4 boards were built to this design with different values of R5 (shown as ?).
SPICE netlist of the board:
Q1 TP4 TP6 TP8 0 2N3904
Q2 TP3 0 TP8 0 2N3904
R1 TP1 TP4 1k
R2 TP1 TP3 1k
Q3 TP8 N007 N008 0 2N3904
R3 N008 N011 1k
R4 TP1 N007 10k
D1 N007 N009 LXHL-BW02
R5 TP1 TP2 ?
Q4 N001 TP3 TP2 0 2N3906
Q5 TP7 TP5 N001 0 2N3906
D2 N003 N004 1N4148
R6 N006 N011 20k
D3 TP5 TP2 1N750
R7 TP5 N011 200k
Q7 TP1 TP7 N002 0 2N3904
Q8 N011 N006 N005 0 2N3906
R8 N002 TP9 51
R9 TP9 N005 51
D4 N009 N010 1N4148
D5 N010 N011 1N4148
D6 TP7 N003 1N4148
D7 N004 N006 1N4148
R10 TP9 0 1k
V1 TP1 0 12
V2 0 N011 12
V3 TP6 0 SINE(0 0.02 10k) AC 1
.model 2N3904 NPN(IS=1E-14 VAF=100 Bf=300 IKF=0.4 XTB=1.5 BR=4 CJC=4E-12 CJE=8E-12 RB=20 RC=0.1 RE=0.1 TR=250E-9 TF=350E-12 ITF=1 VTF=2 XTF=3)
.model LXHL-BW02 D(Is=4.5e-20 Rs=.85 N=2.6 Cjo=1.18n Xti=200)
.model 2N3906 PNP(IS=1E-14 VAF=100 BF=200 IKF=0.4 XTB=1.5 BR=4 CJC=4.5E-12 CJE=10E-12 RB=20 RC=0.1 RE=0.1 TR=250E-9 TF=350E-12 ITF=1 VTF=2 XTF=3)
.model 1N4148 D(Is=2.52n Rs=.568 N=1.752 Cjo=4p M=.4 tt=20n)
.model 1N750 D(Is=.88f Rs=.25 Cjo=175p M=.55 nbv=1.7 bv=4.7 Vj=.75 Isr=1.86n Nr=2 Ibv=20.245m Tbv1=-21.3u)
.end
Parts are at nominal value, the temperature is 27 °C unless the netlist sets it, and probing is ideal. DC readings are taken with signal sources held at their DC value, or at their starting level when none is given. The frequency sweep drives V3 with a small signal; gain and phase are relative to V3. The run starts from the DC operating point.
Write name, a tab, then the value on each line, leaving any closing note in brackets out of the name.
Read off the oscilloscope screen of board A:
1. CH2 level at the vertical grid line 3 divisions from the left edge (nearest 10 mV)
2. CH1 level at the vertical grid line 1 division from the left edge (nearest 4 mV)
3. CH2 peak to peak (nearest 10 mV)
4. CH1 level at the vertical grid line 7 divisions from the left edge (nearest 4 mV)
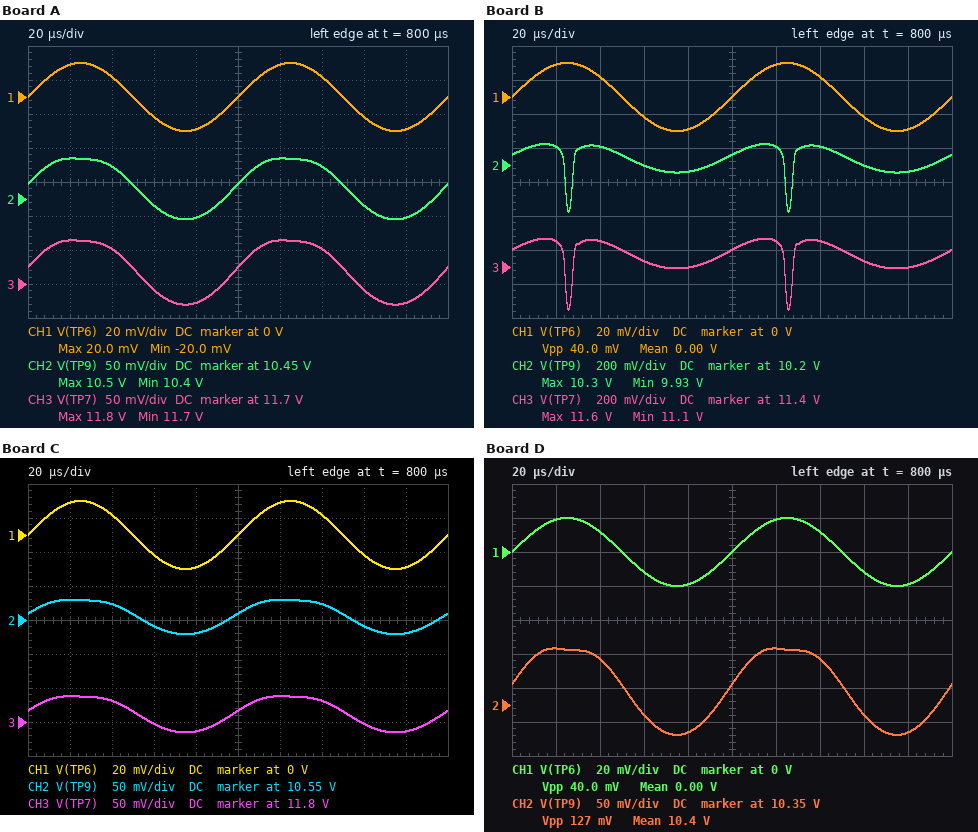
CH2 level at the vertical grid line 3 divisions from the left edge	10.44 V
CH1 level at the vertical grid line 1 division from the left edge	20 mV
CH2 peak to peak	90 mV
CH1 level at the vertical grid line 7 divisions from the left edge	12 mV
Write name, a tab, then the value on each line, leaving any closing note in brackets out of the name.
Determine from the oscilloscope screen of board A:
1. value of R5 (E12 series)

value of R5	120 Ω
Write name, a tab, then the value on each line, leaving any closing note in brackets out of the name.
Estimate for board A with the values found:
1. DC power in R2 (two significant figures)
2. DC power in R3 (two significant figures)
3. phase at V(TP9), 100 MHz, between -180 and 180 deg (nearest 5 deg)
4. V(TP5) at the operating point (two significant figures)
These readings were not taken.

DC power in R2	870 µW
DC power in R3	9.8 mW
phase at V(TP9), 100 MHz, between -180 and 180 deg	-60 deg
V(TP5) at the operating point	11 V
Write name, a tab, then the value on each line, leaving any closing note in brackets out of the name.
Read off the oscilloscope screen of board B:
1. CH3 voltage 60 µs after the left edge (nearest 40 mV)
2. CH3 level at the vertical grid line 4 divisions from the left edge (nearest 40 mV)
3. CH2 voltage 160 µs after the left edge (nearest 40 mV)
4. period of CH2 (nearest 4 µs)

CH3 voltage 60 µs after the left edge	11.44 V
CH3 level at the vertical grid line 4 divisions from the left edge	11.40 V
CH2 voltage 160 µs after the left edge	10.20 V
period of CH2	100 µs
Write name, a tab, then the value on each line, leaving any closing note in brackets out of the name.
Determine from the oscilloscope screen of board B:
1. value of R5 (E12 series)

value of R5	270 Ω
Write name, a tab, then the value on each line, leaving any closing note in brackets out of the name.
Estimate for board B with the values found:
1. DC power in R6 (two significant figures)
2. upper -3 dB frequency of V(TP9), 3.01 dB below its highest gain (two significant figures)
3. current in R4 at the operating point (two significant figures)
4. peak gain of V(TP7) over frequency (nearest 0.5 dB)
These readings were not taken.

DC power in R6	24 mW
upper -3 dB frequency of V(TP9), 3.01 dB below its highest gain	47 MHz
current in R4 at the operating point	2.0 mA
peak gain of V(TP7) over frequency	16.0 dB
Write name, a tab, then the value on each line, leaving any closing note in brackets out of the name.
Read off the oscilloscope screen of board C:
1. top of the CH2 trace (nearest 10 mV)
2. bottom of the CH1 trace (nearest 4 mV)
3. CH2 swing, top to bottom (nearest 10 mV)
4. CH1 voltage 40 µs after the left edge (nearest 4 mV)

top of the CH2 trace	10.58 V
bottom of the CH1 trace	-20 mV
CH2 swing, top to bottom	50 mV
CH1 voltage 40 µs after the left edge	12 mV
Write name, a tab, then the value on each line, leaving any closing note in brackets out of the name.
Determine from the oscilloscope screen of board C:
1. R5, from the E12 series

R5, from the E12 series	68 Ω
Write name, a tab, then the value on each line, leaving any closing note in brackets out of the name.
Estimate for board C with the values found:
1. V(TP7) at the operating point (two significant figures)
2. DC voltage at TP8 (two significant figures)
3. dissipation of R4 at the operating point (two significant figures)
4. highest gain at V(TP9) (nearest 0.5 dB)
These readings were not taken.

V(TP7) at the operating point	12 V
DC voltage at TP8	-660 mV
dissipation of R4 at the operating point	41 mW
highest gain at V(TP9)	5.5 dB
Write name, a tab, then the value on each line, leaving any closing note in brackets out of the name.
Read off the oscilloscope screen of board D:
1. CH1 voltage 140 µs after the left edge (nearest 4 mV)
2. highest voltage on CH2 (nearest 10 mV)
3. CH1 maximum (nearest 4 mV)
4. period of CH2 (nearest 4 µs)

CH1 voltage 140 µs after the left edge	12 mV
highest voltage on CH2	10.43 V
CH1 maximum	20 mV
period of CH2	100 µs
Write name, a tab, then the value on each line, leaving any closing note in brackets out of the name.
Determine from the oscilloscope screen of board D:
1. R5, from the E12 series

R5, from the E12 series	180 Ω
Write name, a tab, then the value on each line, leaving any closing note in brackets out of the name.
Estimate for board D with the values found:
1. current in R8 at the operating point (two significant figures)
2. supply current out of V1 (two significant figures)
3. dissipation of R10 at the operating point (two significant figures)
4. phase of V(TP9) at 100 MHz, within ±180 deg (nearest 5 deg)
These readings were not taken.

current in R8 at the operating point	10 mA
supply current out of V1	17 mA
dissipation of R10 at the operating point	110 mW
phase of V(TP9) at 100 MHz, within ±180 deg	-70 deg
